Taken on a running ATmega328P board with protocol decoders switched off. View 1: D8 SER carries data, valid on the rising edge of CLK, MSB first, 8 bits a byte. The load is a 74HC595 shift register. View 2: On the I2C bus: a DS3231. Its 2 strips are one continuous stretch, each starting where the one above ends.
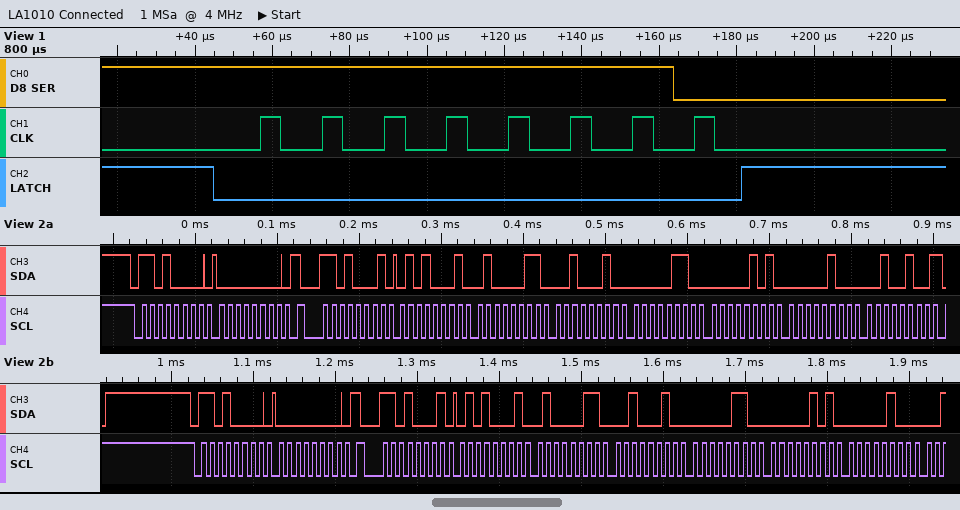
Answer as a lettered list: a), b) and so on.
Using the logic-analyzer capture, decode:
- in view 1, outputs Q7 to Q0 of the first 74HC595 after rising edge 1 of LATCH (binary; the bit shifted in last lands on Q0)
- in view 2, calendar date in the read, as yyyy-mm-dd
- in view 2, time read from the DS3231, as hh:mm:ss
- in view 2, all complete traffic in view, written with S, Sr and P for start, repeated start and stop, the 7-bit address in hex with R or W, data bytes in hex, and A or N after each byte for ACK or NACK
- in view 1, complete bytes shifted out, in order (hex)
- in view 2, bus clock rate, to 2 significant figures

a) 11111110
b) 2024-04-05
c) 22:43:51
d) S 68W A 00 A Sr 68R A 51 A 43 A 22 A 06 A 05 A 04 A 24 N P S 68W A 00 A Sr 68R A 51 A 43 A 22 A 06 A 05 A 04 A
e) 0xFE
f) 100 kHz
